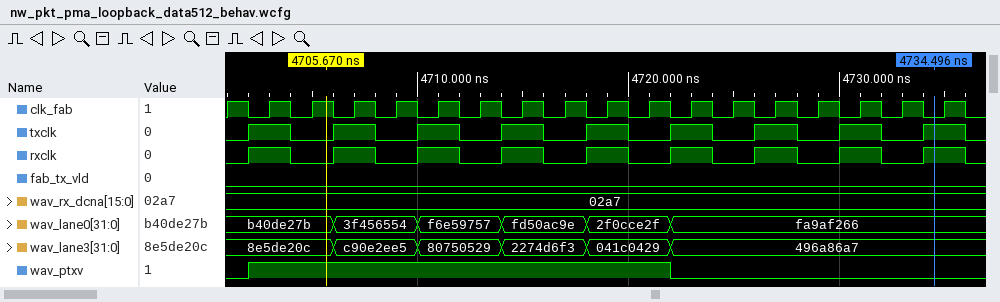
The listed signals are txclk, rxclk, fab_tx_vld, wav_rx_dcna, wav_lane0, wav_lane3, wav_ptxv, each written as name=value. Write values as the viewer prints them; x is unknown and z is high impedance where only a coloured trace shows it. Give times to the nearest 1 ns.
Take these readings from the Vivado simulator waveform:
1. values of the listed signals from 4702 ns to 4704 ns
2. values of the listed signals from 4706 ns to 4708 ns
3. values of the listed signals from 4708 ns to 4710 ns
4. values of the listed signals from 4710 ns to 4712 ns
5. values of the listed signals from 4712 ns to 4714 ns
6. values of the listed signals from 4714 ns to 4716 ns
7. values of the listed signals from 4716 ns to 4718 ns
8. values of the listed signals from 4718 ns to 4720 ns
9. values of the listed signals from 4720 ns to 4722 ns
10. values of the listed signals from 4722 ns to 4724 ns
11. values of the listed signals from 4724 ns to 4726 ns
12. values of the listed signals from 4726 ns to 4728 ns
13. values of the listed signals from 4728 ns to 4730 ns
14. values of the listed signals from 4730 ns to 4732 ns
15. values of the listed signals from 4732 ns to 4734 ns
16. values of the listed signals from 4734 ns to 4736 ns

txclk=1, rxclk=1, fab_tx_vld=0, wav_rx_dcna=02a7, wav_lane0=b40de27b, wav_lane3=8e5de20c, wav_ptxv=1
txclk=1, rxclk=1, fab_tx_vld=0, wav_rx_dcna=02a7, wav_lane0=3f456554, wav_lane3=c90e2ee5, wav_ptxv=1
txclk=0, rxclk=0, fab_tx_vld=0, wav_rx_dcna=02a7, wav_lane0=3f456554, wav_lane3=c90e2ee5, wav_ptxv=1
txclk=1, rxclk=1, fab_tx_vld=0, wav_rx_dcna=02a7, wav_lane0=f6e59757, wav_lane3=80750529, wav_ptxv=1
txclk=0, rxclk=0, fab_tx_vld=0, wav_rx_dcna=02a7, wav_lane0=f6e59757, wav_lane3=80750529, wav_ptxv=1
txclk=1, rxclk=1, fab_tx_vld=0, wav_rx_dcna=02a7, wav_lane0=fd50ac9e, wav_lane3=2274d6f3, wav_ptxv=1
txclk=0, rxclk=0, fab_tx_vld=0, wav_rx_dcna=02a7, wav_lane0=fd50ac9e, wav_lane3=2274d6f3, wav_ptxv=1
txclk=1, rxclk=1, fab_tx_vld=0, wav_rx_dcna=02a7, wav_lane0=2f0cce2f, wav_lane3=041c0429, wav_ptxv=1
txclk=0, rxclk=0, fab_tx_vld=0, wav_rx_dcna=02a7, wav_lane0=2f0cce2f, wav_lane3=041c0429, wav_ptxv=1
txclk=1, rxclk=1, fab_tx_vld=0, wav_rx_dcna=02a7, wav_lane0=fa9af266, wav_lane3=496a86a7, wav_ptxv=0
txclk=0, rxclk=0, fab_tx_vld=0, wav_rx_dcna=02a7, wav_lane0=fa9af266, wav_lane3=496a86a7, wav_ptxv=0
txclk=1, rxclk=1, fab_tx_vld=0, wav_rx_dcna=02a7, wav_lane0=fa9af266, wav_lane3=496a86a7, wav_ptxv=0
txclk=0, rxclk=0, fab_tx_vld=0, wav_rx_dcna=02a7, wav_lane0=fa9af266, wav_lane3=496a86a7, wav_ptxv=0
txclk=1, rxclk=1, fab_tx_vld=0, wav_rx_dcna=02a7, wav_lane0=fa9af266, wav_lane3=496a86a7, wav_ptxv=0
txclk=0, rxclk=0, fab_tx_vld=0, wav_rx_dcna=02a7, wav_lane0=fa9af266, wav_lane3=496a86a7, wav_ptxv=0
txclk=1, rxclk=1, fab_tx_vld=0, wav_rx_dcna=02a7, wav_lane0=fa9af266, wav_lane3=496a86a7, wav_ptxv=0
